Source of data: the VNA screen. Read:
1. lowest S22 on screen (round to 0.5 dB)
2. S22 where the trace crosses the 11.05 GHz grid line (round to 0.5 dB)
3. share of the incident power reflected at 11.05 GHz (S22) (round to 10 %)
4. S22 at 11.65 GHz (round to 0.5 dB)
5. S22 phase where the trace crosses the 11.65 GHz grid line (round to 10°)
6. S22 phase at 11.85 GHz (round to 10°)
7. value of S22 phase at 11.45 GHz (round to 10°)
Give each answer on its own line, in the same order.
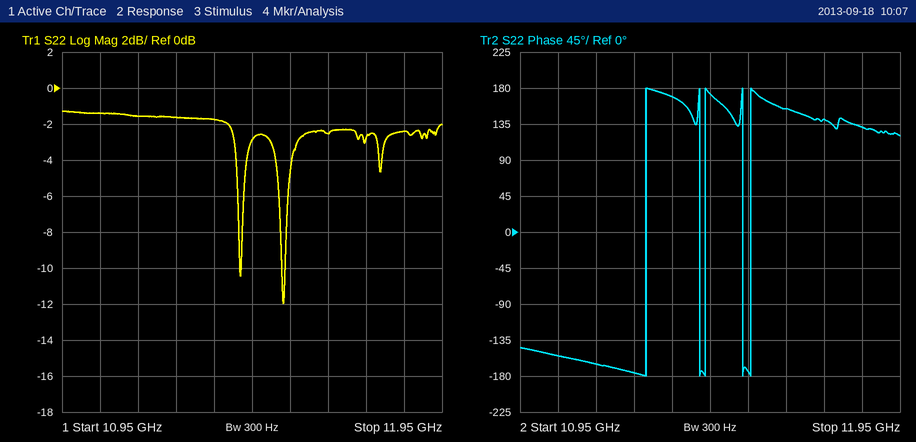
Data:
-12.0 dB
-1.5 dB
70 %
-2.5 dB
150°
130°
170°
